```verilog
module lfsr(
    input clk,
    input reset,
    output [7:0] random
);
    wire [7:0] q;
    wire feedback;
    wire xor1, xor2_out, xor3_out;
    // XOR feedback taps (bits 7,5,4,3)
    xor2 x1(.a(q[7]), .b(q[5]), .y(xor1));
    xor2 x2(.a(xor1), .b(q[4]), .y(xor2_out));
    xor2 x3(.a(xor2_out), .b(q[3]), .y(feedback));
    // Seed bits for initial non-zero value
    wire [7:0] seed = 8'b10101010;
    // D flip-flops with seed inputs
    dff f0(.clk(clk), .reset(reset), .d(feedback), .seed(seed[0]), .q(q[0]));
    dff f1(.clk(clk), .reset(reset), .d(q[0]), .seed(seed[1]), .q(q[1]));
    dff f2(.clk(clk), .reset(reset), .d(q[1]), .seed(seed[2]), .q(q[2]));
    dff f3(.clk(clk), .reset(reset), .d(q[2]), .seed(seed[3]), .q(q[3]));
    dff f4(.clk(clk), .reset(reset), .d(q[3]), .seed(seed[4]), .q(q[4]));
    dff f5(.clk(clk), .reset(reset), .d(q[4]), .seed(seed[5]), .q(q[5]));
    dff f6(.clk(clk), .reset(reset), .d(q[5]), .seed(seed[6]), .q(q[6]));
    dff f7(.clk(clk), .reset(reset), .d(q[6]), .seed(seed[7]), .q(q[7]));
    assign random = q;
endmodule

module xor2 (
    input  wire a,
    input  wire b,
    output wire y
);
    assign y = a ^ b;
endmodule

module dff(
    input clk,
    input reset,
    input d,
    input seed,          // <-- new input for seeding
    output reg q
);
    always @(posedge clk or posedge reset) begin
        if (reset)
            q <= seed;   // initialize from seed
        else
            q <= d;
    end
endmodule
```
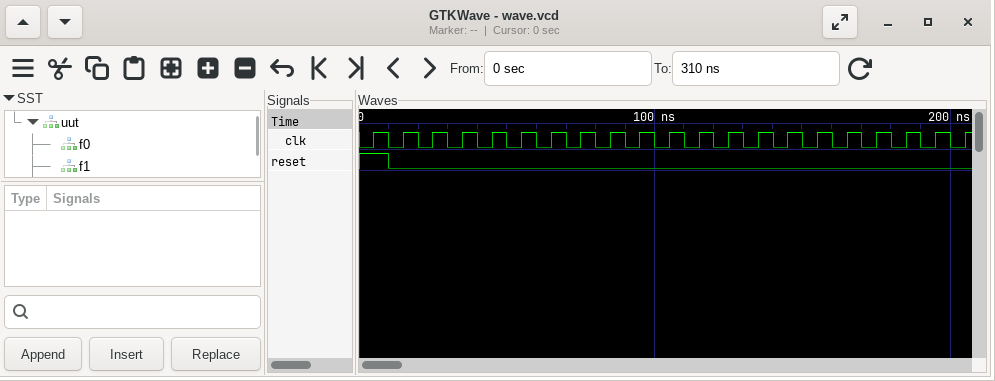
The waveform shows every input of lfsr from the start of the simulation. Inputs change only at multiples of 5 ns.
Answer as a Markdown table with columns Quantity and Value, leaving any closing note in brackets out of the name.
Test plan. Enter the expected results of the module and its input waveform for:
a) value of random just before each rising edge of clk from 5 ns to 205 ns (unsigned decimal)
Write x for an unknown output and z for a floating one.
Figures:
| Quantity | Value |
|---|---|
| value of random just before each rising edge of clk from 5 ns to 205 ns | 170, 170, 85, 171, 87, 175, 95, 190, 124, 249, 242, 229, 202, 148, 40, 80, 161, 66, 132, 9, 19 |
